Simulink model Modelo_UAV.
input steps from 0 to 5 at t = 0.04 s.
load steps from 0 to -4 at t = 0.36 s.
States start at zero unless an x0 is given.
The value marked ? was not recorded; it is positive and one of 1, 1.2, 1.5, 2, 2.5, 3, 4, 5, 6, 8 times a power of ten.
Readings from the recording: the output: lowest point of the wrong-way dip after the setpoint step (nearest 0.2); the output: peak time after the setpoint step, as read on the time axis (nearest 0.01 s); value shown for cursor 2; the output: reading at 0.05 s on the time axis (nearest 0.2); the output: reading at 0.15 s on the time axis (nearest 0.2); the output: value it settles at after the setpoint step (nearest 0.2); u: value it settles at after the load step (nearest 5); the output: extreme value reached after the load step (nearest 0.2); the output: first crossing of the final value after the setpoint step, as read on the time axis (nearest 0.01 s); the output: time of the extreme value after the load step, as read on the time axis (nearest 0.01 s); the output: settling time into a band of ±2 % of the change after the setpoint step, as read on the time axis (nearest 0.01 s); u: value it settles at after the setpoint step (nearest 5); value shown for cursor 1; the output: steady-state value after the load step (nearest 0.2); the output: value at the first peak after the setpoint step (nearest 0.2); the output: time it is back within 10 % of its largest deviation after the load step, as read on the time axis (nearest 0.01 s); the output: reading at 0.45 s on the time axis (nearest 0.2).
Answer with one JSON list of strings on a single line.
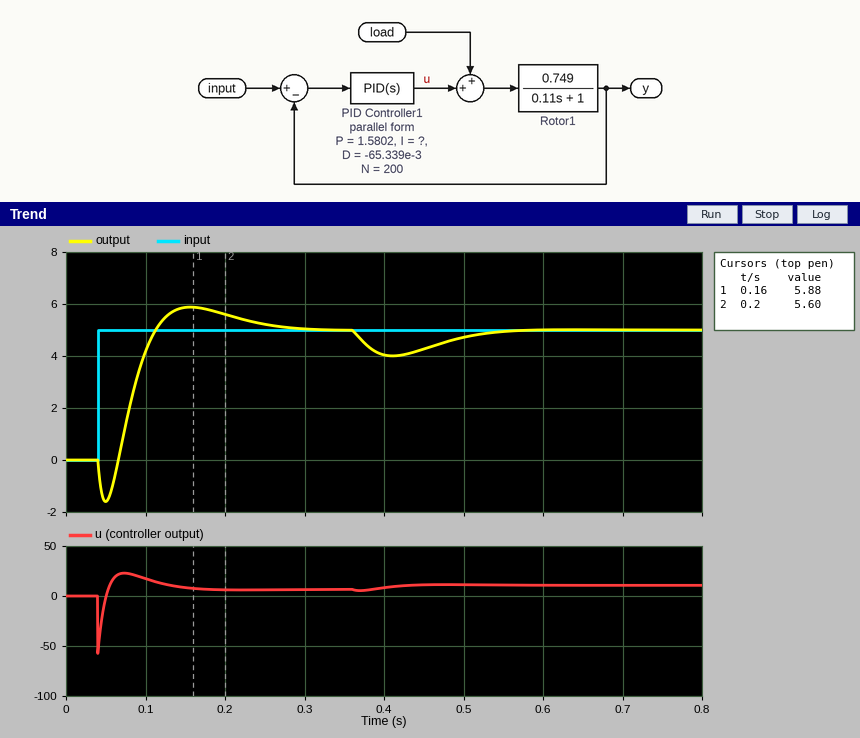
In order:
["-1.6", "0.16 s", "5.60", "-1.6", "5.8", "5.0", "10", "4.0", "0.11 s", "0.41 s", "0.28 s", "5", "5.88", "5.0", "5.8", "0.54 s", "4.2"]
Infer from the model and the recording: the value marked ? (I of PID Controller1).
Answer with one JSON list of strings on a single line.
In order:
["40"]
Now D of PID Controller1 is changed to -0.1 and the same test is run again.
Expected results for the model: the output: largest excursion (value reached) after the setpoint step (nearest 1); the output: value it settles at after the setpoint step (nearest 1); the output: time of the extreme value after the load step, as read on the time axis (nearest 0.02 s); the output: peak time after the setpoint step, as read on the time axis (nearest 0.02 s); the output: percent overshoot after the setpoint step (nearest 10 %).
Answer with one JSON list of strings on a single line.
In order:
["7", "5", "0.40 s", "0.12 s", "40 %"]
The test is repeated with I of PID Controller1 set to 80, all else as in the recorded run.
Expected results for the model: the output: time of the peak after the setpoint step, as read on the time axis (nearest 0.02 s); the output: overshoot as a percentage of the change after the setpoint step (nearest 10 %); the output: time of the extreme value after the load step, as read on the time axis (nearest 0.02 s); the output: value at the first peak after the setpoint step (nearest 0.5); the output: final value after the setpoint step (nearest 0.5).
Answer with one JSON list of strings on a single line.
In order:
["0.12 s", "40 %", "0.40 s", "7.0", "5.0"]
